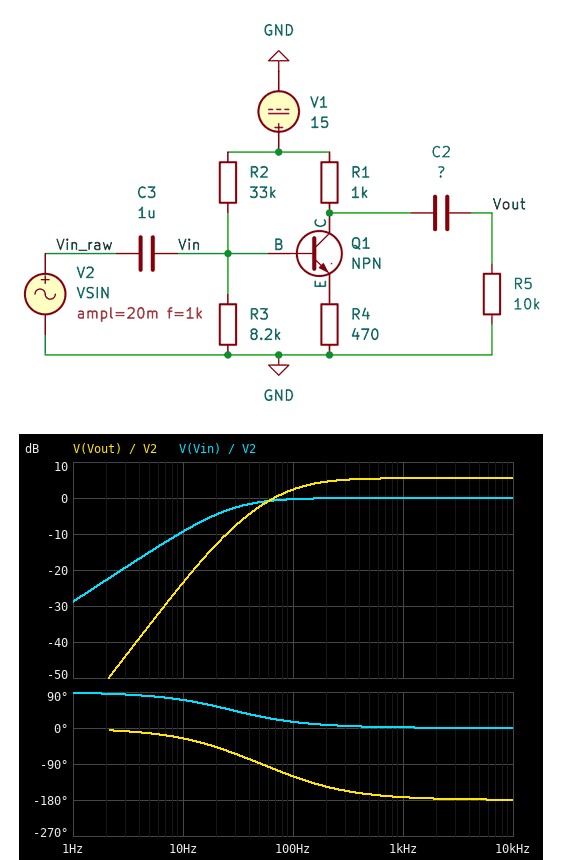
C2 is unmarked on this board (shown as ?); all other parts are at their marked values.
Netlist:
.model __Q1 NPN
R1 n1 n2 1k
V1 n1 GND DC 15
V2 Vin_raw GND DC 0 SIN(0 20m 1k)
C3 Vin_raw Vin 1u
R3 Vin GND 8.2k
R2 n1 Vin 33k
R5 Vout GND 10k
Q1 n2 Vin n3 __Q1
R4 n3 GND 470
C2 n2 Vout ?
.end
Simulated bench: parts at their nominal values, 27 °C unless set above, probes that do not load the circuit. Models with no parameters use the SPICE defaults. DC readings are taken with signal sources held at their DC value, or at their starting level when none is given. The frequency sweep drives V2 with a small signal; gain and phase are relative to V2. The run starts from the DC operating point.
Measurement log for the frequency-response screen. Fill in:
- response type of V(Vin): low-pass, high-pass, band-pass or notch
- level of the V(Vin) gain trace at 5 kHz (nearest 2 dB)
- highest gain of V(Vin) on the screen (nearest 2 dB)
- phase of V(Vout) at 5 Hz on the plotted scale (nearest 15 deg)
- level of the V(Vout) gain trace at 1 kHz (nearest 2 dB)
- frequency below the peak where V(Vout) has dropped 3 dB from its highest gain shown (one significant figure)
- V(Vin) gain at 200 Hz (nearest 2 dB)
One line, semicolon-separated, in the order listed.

high-pass; 0 dB; 0 dB; -15 deg; 6 dB; 100 Hz; 0 dB
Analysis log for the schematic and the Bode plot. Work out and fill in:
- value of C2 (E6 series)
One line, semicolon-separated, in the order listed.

150 nF
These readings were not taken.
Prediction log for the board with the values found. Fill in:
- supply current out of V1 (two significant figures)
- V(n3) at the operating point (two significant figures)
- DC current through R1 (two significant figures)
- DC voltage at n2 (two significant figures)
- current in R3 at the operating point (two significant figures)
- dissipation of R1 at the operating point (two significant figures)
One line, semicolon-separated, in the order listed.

4.4 mA; 1.9 V; 4.0 mA; 11 V; 330 µA; 16 mW
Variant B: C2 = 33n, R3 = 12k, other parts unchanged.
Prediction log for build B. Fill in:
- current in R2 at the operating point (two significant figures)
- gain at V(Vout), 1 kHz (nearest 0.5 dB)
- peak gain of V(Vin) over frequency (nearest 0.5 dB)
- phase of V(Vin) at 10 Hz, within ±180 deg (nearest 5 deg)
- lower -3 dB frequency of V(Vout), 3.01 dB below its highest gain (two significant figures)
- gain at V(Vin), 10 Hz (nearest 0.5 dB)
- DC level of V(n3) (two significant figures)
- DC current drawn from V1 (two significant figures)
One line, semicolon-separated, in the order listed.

350 µA; 5.0 dB; 0 dB; 65 deg; 440 Hz; -7.5 dB; 2.7 V; 6.0 mA
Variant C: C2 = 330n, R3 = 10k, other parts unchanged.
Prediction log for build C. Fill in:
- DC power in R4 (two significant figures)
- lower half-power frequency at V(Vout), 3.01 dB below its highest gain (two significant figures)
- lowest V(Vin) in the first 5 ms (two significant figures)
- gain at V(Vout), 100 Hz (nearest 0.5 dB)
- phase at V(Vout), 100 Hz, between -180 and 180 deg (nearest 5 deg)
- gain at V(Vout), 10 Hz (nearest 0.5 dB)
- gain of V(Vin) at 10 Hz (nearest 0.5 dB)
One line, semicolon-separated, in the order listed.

11 mW; 54 Hz; 3.1 V; 4.5 dB; -145 deg; -16.0 dB; -8.5 dB
